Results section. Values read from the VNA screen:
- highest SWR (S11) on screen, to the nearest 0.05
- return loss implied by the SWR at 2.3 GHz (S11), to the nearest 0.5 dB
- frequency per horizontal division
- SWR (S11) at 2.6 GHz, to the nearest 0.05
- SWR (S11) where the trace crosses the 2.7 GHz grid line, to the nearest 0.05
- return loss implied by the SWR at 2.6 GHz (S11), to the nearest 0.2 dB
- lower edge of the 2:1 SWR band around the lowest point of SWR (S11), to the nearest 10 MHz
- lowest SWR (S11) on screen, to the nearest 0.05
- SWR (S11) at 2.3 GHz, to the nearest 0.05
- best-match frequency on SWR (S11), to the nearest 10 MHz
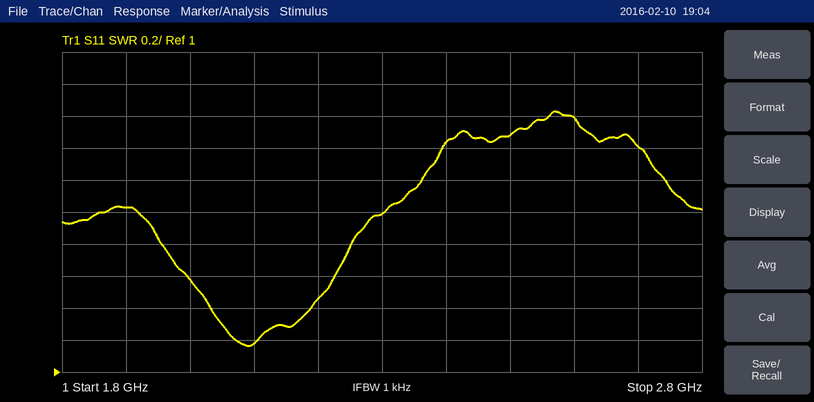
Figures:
2.65
9.5 dB
100 MHz
2.60
2.40
7.0 dB
1.92 GHz
1.15
2.00
2.09 GHz
